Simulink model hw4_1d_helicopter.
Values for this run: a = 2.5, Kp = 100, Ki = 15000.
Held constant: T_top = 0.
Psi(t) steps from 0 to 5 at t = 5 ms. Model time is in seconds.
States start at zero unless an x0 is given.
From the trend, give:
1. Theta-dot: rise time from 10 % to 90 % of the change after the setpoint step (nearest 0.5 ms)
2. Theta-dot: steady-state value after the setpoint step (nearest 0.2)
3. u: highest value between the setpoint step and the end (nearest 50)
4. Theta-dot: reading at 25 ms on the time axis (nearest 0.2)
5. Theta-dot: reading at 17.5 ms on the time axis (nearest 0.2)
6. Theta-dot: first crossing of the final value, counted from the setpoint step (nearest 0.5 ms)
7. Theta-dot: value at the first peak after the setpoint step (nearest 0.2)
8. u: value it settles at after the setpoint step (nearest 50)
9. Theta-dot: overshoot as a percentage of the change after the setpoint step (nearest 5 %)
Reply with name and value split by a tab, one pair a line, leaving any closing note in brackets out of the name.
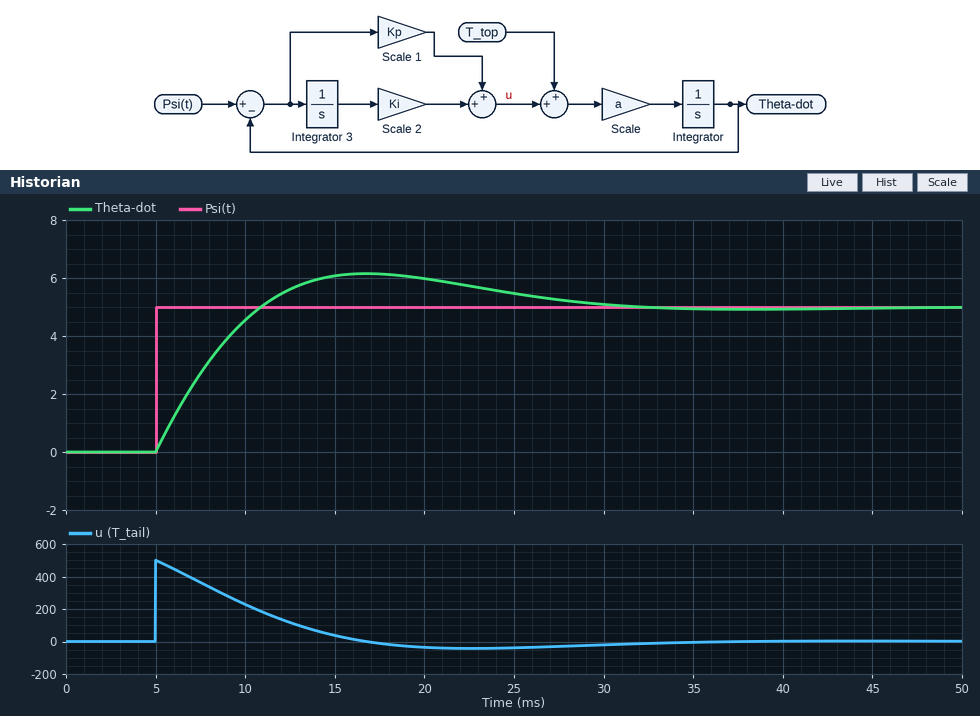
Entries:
Theta-dot: rise time from 10 % to 90 % of the change after the setpoint step	4.5 ms
Theta-dot: steady-state value after the setpoint step	5.0
u: highest value between the setpoint step and the end	500
Theta-dot: reading at 25 ms on the time axis	5.4
Theta-dot: reading at 17.5 ms on the time axis	6.2
Theta-dot: first crossing of the final value, counted from the setpoint step	6.0 ms
Theta-dot: value at the first peak after the setpoint step	6.2
u: value it settles at after the setpoint step	0
Theta-dot: overshoot as a percentage of the change after the setpoint step	25 %
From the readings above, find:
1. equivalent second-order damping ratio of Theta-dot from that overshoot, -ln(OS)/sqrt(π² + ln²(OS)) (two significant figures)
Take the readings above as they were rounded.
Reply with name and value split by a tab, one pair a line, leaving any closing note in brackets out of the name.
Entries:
equivalent second-order damping ratio of Theta-dot from that overshoot, -ln(OS)/sqrt(π² + ln²(OS))	0.40
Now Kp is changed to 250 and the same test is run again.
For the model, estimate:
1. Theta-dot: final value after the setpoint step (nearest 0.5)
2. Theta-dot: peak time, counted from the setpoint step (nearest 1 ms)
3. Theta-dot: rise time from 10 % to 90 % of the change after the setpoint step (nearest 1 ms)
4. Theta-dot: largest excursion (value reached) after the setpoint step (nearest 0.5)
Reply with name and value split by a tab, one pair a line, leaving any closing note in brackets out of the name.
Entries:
Theta-dot: final value after the setpoint step	5.0
Theta-dot: peak time, counted from the setpoint step	9 ms
Theta-dot: rise time from 10 % to 90 % of the change after the setpoint step	3 ms
Theta-dot: largest excursion (value reached) after the setpoint step	5.5
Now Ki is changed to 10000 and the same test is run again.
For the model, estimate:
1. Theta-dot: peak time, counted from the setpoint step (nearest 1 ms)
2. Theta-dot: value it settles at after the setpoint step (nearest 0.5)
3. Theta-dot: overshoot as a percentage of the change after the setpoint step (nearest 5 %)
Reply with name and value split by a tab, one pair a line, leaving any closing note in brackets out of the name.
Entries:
Theta-dot: peak time, counted from the setpoint step	14 ms
Theta-dot: value it settles at after the setpoint step	5.0
Theta-dot: overshoot as a percentage of the change after the setpoint step	20 %
